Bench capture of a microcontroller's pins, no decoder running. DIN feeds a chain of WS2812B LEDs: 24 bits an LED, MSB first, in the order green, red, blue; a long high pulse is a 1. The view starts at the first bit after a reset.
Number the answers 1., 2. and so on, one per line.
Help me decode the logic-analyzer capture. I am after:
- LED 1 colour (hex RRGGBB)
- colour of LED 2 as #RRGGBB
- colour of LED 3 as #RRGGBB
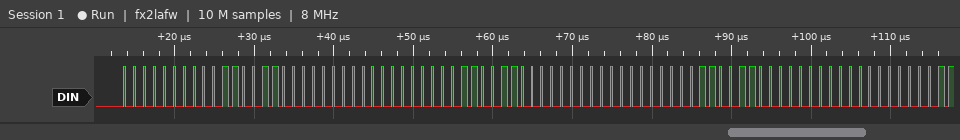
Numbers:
1. #330000
2. #330000
3. #330000
